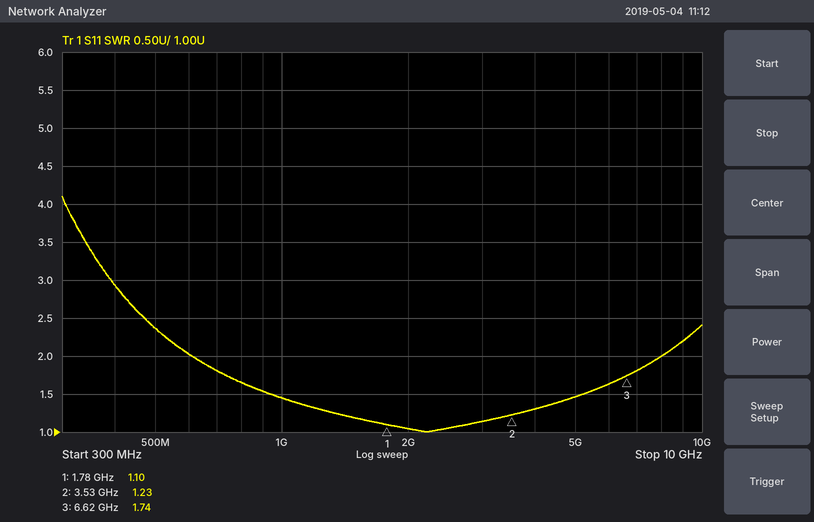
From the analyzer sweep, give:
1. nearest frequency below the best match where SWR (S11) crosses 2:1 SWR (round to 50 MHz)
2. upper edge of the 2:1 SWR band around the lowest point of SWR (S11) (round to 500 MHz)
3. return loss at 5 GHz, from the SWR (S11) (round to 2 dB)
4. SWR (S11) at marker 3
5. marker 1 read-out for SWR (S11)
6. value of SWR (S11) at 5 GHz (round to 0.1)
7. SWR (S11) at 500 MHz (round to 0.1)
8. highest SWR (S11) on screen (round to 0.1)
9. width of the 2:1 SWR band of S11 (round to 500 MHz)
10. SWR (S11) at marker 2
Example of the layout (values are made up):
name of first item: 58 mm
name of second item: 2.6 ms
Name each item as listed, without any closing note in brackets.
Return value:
nearest frequency below the best match where SWR (S11) crosses 2:1 SWR: 600 MHz
upper edge of the 2:1 SWR band around the lowest point of SWR (S11): 8.0 GHz
return loss at 5 GHz, from the SWR (S11): 14 dB
SWR (S11) at marker 3: 1.74
marker 1 read-out for SWR: 1.10
value of SWR (S11) at 5 GHz: 1.5
SWR (S11) at 500 MHz: 2.4
highest SWR (S11) on screen: 4.1
width of the 2:1 SWR band of S11: 7.5 GHz
SWR (S11) at marker 2: 1.23
